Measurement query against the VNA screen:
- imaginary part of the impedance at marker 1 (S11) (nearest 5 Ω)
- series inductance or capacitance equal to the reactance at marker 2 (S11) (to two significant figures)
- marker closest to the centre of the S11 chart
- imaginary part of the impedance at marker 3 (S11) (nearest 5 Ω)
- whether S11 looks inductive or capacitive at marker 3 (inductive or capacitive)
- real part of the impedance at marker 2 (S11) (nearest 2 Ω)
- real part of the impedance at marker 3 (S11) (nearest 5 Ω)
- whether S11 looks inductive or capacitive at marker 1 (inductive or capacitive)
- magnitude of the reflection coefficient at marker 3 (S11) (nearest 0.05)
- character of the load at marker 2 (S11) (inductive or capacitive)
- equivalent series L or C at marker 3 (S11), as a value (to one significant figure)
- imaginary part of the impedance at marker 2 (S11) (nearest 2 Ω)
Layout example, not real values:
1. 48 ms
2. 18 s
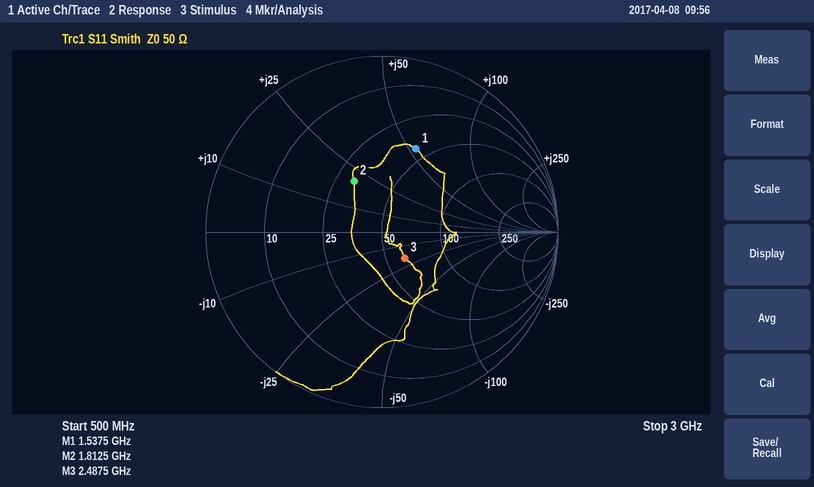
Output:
1. +55 Ω
2. 1.8 nH
3. marker 3
4. -20 Ω
5. capacitive
6. 32 Ω
7. 60 Ω
8. inductive
9. 0.20
10. inductive
11. 3 pF
12. +20 Ω
